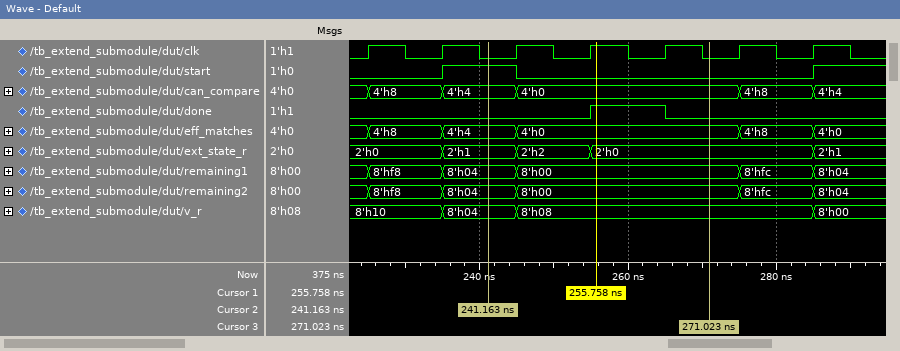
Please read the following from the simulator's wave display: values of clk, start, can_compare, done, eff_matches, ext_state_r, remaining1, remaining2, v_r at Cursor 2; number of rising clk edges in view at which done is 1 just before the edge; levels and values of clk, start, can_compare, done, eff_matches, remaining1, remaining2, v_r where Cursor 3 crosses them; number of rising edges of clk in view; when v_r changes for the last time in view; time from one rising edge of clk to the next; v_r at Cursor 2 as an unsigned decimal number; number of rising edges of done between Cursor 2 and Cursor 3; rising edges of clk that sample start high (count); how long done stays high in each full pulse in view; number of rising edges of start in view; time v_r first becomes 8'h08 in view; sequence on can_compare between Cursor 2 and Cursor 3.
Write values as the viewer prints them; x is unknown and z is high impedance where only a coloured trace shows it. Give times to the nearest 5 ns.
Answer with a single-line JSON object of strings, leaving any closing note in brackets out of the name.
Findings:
{"values of clk, start, can_compare, done, eff_matches, ext_state_r, remaining1, remaining2, v_r at Cursor 2": "clk=0, start=1, can_compare=4'h4, done=0, eff_matches=4'h4, ext_state_r=2'h1, remaining1=8'h04, remaining2=8'h04, v_r=8'h04", "number of rising clk edges in view at which done is 1 just before the edge": "1", "levels and values of clk, start, can_compare, done, eff_matches, remaining1, remaining2, v_r where Cursor 3 crosses them": "clk=0, start=0, can_compare=4'h0, done=0, eff_matches=4'h0, remaining1=8'h00, remaining2=8'h00, v_r=8'h08", "number of rising edges of clk in view": "7", "when v_r changes for the last time in view": "285 ns", "time from one rising edge of clk to the next": "10 ns", "v_r at Cursor 2 as an unsigned decimal number": "4", "number of rising edges of done between Cursor 2 and Cursor 3": "1", "rising edges of clk that sample start high": "1", "how long done stays high in each full pulse in view": "10 ns", "number of rising edges of start in view": "2", "time v_r first becomes 8'h08 in view": "245 ns", "sequence on can_compare between Cursor 2 and Cursor 3": "4'h4, 4'h0"}
